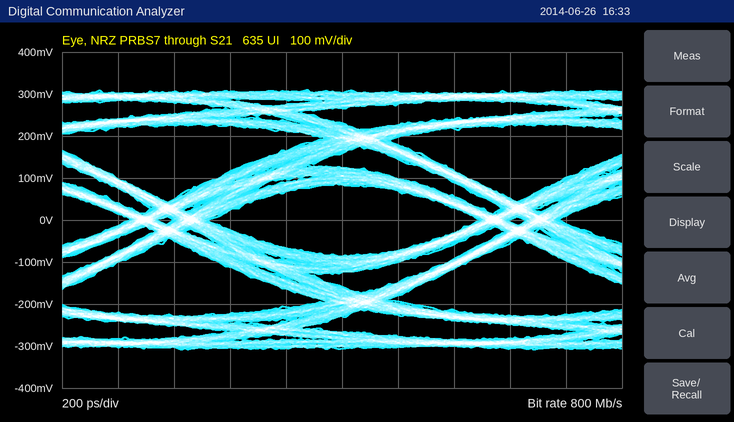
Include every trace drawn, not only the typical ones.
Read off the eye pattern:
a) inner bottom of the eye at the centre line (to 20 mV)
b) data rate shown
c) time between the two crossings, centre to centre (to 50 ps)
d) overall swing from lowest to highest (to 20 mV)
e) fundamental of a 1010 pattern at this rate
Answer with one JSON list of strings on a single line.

["-80 mV", "800 Mb/s", "1.25 ns", "620 mV", "400 MHz"]
